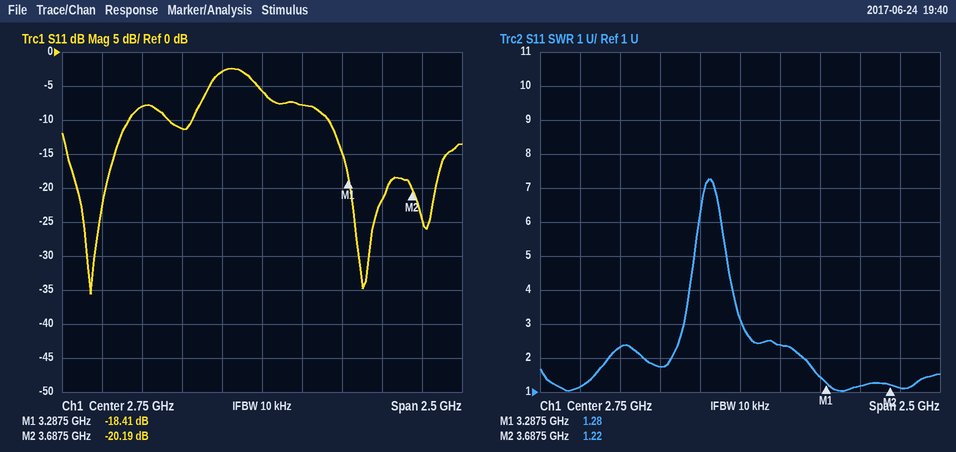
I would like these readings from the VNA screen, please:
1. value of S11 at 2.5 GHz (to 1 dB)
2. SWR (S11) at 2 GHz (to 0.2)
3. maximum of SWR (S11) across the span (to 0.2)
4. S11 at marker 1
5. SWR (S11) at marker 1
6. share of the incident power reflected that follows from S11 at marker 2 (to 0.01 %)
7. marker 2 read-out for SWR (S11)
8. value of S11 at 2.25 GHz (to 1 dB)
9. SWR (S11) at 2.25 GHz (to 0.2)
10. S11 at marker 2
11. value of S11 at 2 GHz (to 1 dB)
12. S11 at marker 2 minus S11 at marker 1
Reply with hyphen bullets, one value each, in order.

- -3 dB
- 2.4
- 7.2
- -18.41 dB
- 1.28
- 0.96 %
- 1.22
- -11 dB
- 1.8
- -20.19 dB
- -8 dB
- -1.78 dB
